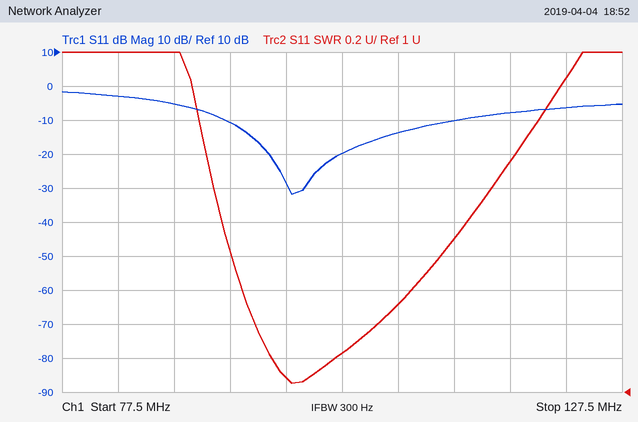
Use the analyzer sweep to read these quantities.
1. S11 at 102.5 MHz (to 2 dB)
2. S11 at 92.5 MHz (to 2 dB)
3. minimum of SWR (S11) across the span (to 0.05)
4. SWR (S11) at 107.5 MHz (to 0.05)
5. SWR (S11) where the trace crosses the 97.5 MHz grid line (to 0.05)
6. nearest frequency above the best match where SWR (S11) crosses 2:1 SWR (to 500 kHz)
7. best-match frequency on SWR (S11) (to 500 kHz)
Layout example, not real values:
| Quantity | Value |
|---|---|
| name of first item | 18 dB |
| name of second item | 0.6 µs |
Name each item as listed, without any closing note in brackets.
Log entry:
| Quantity | Value |
|---|---|
| S11 at 102.5 MHz | -20 dB |
| S11 at 92.5 MHz | -10 dB |
| minimum of SWR (S11) across the span | 1.05 |
| SWR (S11) at 107.5 MHz | 1.50 |
| SWR (S11) where the trace crosses the 97.5 MHz grid line | 1.10 |
| nearest frequency above the best match where SWR (S11) crosses 2:1 SWR | 113.5 MHz |
| best-match frequency on SWR (S11) | 98.0 MHz |
